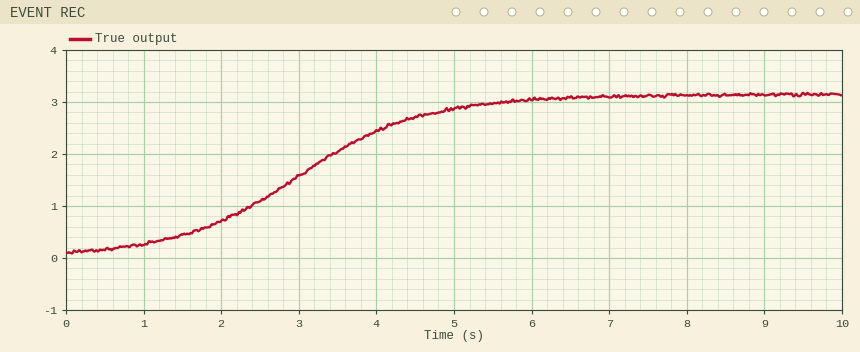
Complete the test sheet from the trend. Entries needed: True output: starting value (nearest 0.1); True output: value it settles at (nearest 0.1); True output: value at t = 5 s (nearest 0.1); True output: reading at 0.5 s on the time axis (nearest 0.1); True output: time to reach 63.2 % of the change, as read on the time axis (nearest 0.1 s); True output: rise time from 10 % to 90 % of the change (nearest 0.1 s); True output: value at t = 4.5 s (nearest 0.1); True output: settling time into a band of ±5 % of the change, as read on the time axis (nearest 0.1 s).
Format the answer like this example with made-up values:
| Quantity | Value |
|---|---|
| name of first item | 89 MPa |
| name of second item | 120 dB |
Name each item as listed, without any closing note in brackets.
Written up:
| Quantity | Value |
|---|---|
| True output: starting value | 0.1 |
| True output: value it settles at | 3.1 |
| True output: value at t = 5 s | 2.9 |
| True output: reading at 0.5 s on the time axis | 0.2 |
| True output: time to reach 63.2 % of the change, as read on the time axis | 3.5 s |
| True output: rise time from 10 % to 90 % of the change | 3.5 s |
| True output: value at t = 4.5 s | 2.7 |
| True output: settling time into a band of ±5 % of the change, as read on the time axis | 5.6 s |
